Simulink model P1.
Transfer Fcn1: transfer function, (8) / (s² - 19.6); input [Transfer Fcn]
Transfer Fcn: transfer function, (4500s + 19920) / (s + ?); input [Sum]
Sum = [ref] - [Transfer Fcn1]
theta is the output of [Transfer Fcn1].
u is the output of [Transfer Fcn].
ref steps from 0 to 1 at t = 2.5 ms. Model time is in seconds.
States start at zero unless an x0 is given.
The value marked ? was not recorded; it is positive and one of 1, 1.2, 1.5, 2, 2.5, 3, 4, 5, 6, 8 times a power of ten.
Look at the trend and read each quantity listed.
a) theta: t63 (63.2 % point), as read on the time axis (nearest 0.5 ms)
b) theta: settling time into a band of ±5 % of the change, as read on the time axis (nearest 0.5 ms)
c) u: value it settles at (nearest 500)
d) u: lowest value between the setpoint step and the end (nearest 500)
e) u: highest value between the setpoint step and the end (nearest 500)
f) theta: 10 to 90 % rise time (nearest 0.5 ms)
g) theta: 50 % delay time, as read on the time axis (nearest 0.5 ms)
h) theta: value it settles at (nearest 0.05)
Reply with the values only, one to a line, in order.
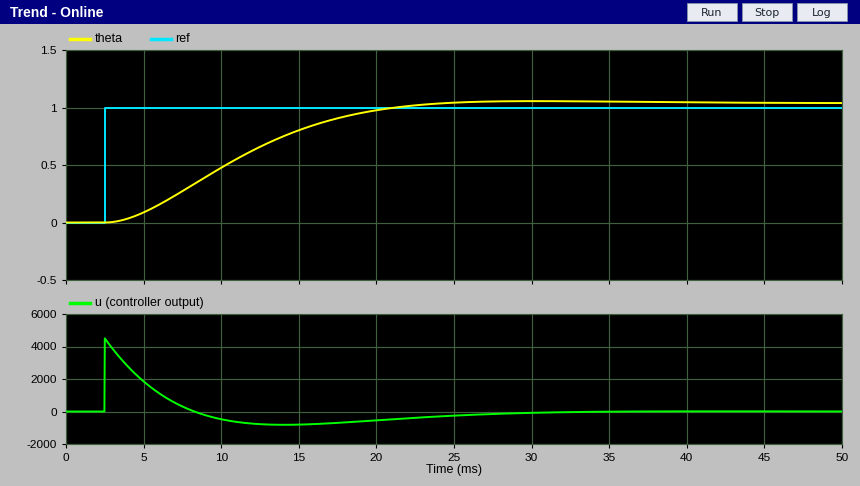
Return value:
12.5 ms
20.5 ms
0
-1000
4500
13.0 ms
10.5 ms
1.05
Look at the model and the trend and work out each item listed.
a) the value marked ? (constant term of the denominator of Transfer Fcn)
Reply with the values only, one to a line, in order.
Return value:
300
